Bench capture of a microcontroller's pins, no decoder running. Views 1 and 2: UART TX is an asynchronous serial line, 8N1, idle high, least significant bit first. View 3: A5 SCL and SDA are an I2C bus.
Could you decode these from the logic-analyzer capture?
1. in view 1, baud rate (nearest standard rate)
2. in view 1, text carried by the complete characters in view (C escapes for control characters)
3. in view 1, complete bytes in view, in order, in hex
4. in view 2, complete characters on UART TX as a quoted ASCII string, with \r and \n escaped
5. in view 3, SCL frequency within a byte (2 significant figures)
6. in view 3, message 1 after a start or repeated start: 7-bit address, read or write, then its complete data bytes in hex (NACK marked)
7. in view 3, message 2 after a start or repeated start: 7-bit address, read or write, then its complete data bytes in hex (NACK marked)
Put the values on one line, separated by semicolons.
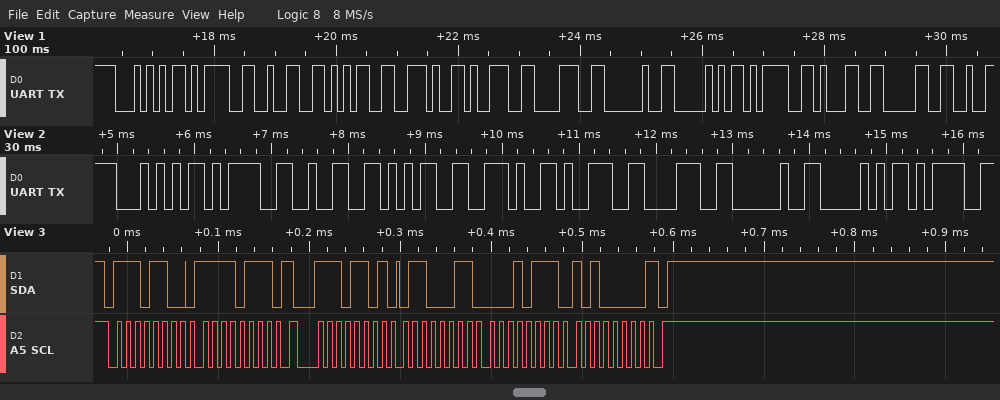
9600 baud; "T=25.98 P=10"; 54 3D 32 35 2E 39 38 20 50 3D 31 30; "T=25.98 P="; 100 kHz; 0x76 write: F7; 0x76 read: 63 17 A0 NACK
